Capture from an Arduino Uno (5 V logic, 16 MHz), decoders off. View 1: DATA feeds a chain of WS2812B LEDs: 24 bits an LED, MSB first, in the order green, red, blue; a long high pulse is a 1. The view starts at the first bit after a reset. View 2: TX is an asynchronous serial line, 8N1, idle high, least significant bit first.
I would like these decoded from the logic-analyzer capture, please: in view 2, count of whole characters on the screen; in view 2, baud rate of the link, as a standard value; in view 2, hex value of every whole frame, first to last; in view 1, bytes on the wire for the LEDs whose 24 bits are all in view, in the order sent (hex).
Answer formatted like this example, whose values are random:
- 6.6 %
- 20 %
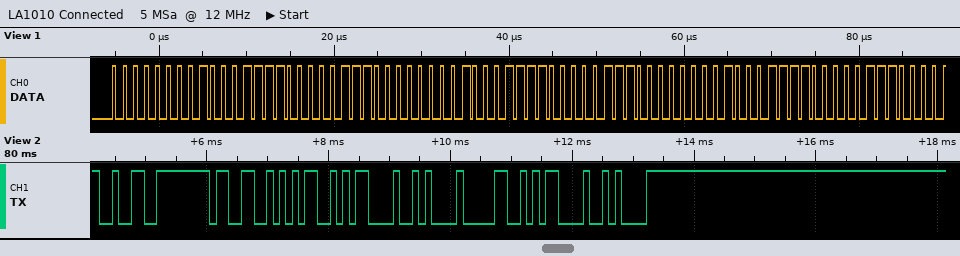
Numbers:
- 8
- 9600 baud
- 32 33 35 0D 0A 30 0D 0A
- 00 8F 07 00 8F 07 00 8F 07
